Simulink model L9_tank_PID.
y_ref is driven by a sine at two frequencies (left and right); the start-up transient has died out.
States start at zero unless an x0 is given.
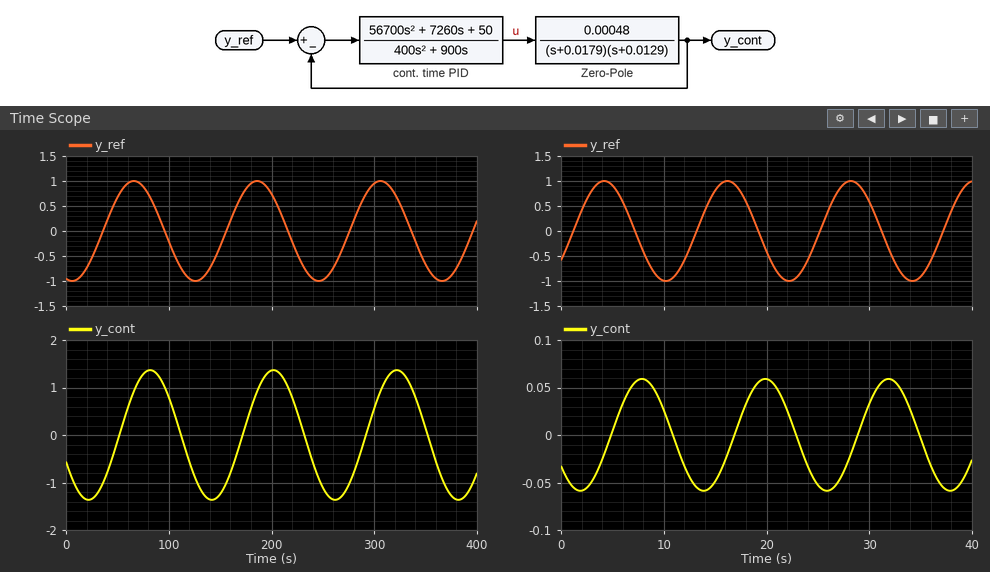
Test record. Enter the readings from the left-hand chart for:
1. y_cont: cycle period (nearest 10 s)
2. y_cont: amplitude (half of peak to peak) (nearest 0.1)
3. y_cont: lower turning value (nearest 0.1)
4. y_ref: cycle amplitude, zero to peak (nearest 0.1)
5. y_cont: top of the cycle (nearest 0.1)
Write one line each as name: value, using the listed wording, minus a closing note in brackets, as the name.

y_cont: cycle period: 120 s
y_cont: amplitude (half of peak to peak): 1.4
y_cont: lower turning value: -1.4
y_ref: cycle amplitude, zero to peak: 1.0
y_cont: top of the cycle: 1.4
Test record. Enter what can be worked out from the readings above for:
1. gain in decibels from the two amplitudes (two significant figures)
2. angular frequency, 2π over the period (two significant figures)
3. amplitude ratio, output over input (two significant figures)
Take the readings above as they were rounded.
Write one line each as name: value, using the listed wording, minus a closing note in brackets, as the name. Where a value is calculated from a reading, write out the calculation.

gain in decibels from the two amplitudes: 20 log10(1.4 / 1) = 2.9 dB
angular frequency, 2π over the period: 2π / 120 = 0.052 rad/s
amplitude ratio, output over input: 1.4 / 1 = 1.4
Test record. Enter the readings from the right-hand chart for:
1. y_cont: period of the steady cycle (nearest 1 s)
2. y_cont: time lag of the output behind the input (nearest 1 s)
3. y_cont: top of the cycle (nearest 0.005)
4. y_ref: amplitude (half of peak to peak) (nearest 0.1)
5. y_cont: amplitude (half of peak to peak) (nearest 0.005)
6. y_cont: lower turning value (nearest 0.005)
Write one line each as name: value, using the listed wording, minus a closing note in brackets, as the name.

y_cont: period of the steady cycle: 12 s
y_cont: time lag of the output behind the input: 4 s
y_cont: top of the cycle: 0.060
y_ref: amplitude (half of peak to peak): 1.0
y_cont: amplitude (half of peak to peak): 0.060
y_cont: lower turning value: -0.060
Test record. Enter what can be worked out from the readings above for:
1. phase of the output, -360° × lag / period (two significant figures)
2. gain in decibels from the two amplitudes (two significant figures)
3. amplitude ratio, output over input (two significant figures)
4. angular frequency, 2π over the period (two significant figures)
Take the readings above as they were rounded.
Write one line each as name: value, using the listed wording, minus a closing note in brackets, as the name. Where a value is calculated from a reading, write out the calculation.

phase of the output, -360° × lag / period: -360 × 4 / 12 = -120°
gain in decibels from the two amplitudes: 20 log10(0.06 / 1) = -24 dB
amplitude ratio, output over input: 0.06 / 1 = 0.060
angular frequency, 2π over the period: 2π / 12 = 0.52 rad/s
